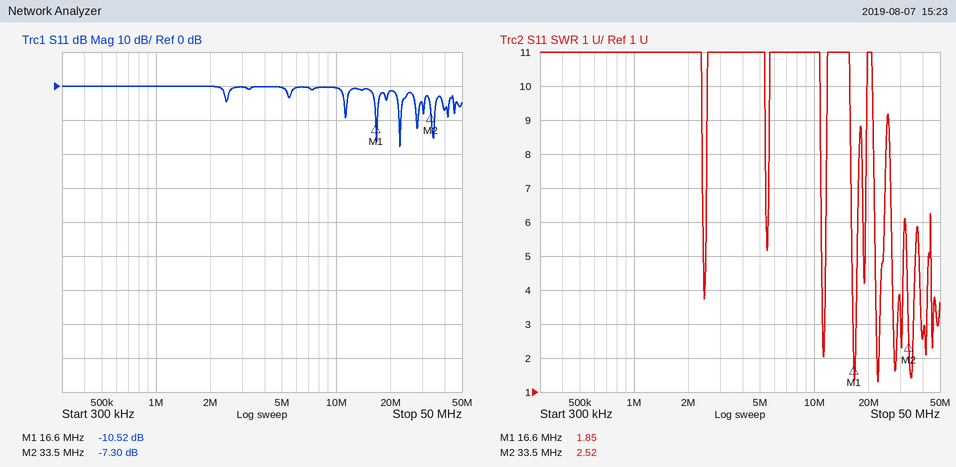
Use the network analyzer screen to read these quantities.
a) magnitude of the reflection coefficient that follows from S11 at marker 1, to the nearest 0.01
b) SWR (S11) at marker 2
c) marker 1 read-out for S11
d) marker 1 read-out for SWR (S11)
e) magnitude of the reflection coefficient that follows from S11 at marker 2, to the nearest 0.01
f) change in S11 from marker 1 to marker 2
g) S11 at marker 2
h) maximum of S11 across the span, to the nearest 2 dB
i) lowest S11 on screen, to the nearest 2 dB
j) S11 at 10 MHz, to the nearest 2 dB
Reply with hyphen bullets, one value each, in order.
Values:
- 0.30
- 2.52
- -10.52 dB
- 1.85
- 0.43
- 3.22 dB
- -7.30 dB
- 0 dB
- -18 dB
- 0 dB
